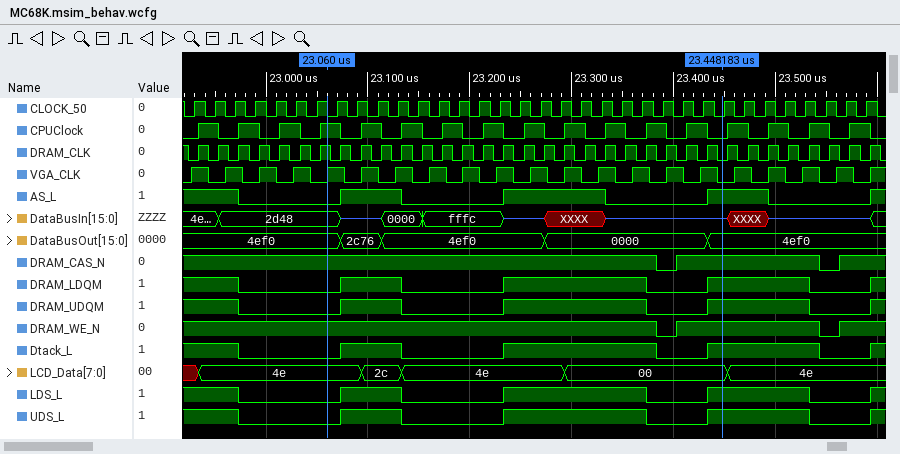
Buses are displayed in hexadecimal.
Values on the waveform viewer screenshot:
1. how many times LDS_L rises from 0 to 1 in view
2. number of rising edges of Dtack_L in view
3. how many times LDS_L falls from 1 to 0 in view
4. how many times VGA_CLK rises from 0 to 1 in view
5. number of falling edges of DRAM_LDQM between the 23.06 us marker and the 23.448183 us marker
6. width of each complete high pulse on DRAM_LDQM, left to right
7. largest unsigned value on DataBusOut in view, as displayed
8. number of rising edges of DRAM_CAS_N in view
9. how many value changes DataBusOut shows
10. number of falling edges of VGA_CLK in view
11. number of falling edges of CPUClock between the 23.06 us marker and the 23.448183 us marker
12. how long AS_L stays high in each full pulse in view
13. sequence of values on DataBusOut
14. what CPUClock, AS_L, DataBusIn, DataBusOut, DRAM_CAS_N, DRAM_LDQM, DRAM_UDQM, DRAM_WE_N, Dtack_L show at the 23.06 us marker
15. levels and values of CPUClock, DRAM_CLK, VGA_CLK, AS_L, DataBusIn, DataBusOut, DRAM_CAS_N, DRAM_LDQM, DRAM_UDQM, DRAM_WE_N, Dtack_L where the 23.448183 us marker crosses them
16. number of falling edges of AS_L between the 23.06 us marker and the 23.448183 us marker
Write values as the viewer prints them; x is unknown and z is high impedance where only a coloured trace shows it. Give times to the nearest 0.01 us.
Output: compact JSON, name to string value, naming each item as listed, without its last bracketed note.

{"how many times LDS_L rises from 0 to 1 in view": "4", "number of rising edges of Dtack_L in view": "4", "how many times LDS_L falls from 1 to 0 in view": "4", "how many times VGA_CLK rises from 0 to 1 in view": "21", "number of falling edges of DRAM_LDQM between the 23.06 us marker and the 23.448183 us marker": "2", "width of each complete high pulse on DRAM_LDQM, left to right": "0.06 us, 0.14 us, 0.1 us", "largest unsigned value on DataBusOut in view, as displayed": "4ef0", "number of rising edges of DRAM_CAS_N in view": "2", "how many value changes DataBusOut shows": "4", "number of falling edges of VGA_CLK in view": "20", "number of falling edges of CPUClock between the 23.06 us marker and the 23.448183 us marker": "10", "how long AS_L stays high in each full pulse in view": "0.06 us, 0.1 us, 0.06 us", "sequence of values on DataBusOut": "4ef0, 2c76, 4ef0, 0000, 4ef0", "what CPUClock, AS_L, DataBusIn, DataBusOut, DRAM_CAS_N, DRAM_LDQM, DRAM_UDQM, DRAM_WE_N, Dtack_L show at the 23.06 us marker": "CPUClock=1, AS_L=0, DataBusIn=2d48, DataBusOut=4ef0, DRAM_CAS_N=1, DRAM_LDQM=0, DRAM_UDQM=0, DRAM_WE_N=1, Dtack_L=0", "levels and values of CPUClock, DRAM_CLK, VGA_CLK, AS_L, DataBusIn, DataBusOut, DRAM_CAS_N, DRAM_LDQM, DRAM_UDQM, DRAM_WE_N, Dtack_L where the 23.448183 us marker crosses them": "CPUClock=0, DRAM_CLK=0, VGA_CLK=0, AS_L=1, DataBusIn=z, DataBusOut=4ef0, DRAM_CAS_N=1, DRAM_LDQM=1, DRAM_UDQM=1, DRAM_WE_N=1, Dtack_L=1", "number of falling edges of AS_L between the 23.06 us marker and the 23.448183 us marker": "2"}
